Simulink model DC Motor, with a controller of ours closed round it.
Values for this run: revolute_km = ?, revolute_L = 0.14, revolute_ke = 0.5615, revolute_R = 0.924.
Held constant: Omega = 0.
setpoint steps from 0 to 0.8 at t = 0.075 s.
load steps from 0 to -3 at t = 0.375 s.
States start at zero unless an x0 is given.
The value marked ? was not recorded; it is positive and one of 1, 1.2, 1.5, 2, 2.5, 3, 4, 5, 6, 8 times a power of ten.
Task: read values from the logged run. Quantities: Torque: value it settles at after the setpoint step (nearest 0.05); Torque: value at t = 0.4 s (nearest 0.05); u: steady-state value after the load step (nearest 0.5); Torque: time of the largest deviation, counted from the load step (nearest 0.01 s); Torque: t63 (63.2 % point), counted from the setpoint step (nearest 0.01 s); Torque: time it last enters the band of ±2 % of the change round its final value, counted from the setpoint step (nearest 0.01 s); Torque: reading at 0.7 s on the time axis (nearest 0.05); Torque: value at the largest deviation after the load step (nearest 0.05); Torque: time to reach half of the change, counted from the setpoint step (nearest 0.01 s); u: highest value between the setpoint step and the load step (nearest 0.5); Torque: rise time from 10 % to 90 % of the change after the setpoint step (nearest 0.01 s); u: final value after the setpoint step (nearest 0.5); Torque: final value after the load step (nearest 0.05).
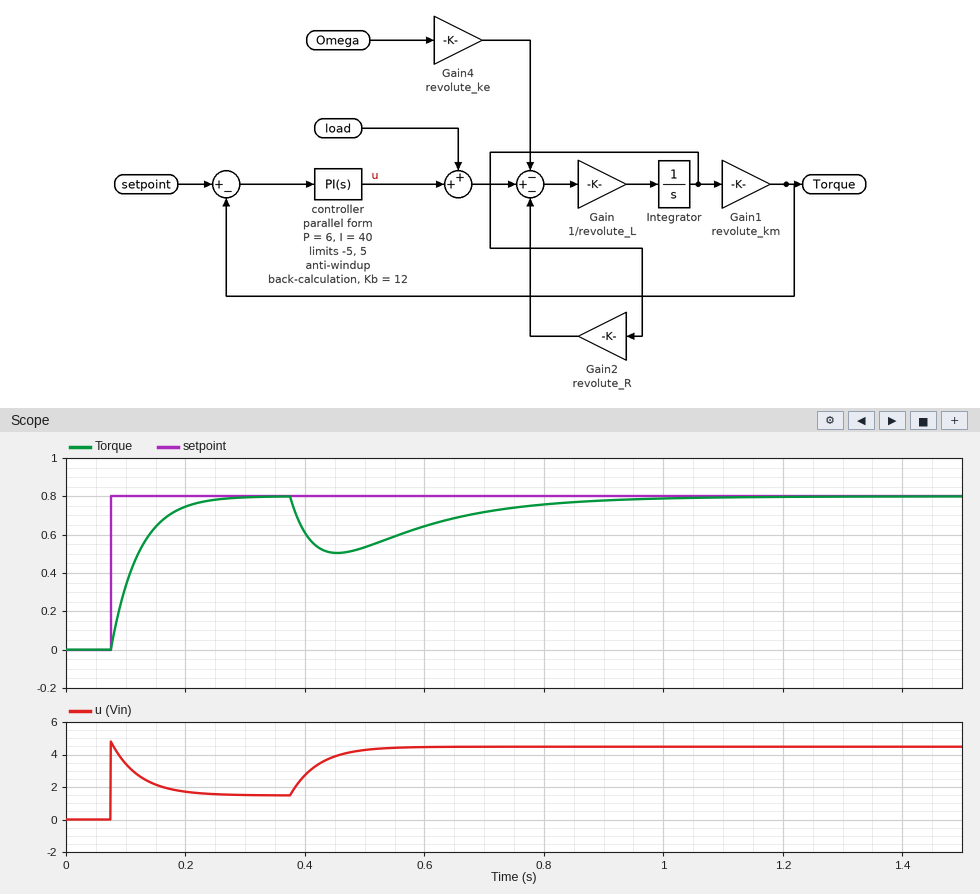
0.80
0.60
4.5
0.08 s
0.05 s
0.18 s
0.70
0.50
0.03 s
5.0
0.10 s
1.5
0.80
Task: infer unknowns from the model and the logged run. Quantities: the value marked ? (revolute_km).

0.5
